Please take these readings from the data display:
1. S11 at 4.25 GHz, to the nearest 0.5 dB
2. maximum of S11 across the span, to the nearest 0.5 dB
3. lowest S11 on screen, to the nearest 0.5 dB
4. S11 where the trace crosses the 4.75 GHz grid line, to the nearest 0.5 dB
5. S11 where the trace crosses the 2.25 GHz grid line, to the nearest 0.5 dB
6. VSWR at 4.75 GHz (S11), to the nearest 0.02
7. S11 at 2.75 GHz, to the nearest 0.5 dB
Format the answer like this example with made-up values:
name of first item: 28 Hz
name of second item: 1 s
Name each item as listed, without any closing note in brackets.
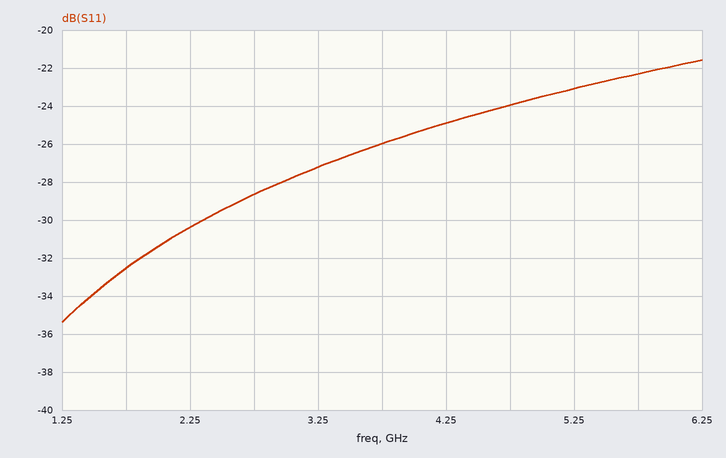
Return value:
S11 at 4.25 GHz, to the nearest 0.5 dB: -25.0 dB
maximum of S11 across the span, to the nearest 0.5 dB: -21.5 dB
lowest S11 on screen, to the nearest 0.5 dB: -35.5 dB
S11 where the trace crosses the 4.75 GHz grid line, to the nearest 0.5 dB: -24.0 dB
S11 where the trace crosses the 2.25 GHz grid line, to the nearest 0.5 dB: -30.5 dB
VSWR at 4.75 GHz (S11), to the nearest 0.02: 1.14
S11 at 2.75 GHz, to the nearest 0.5 dB: -28.5 dB
